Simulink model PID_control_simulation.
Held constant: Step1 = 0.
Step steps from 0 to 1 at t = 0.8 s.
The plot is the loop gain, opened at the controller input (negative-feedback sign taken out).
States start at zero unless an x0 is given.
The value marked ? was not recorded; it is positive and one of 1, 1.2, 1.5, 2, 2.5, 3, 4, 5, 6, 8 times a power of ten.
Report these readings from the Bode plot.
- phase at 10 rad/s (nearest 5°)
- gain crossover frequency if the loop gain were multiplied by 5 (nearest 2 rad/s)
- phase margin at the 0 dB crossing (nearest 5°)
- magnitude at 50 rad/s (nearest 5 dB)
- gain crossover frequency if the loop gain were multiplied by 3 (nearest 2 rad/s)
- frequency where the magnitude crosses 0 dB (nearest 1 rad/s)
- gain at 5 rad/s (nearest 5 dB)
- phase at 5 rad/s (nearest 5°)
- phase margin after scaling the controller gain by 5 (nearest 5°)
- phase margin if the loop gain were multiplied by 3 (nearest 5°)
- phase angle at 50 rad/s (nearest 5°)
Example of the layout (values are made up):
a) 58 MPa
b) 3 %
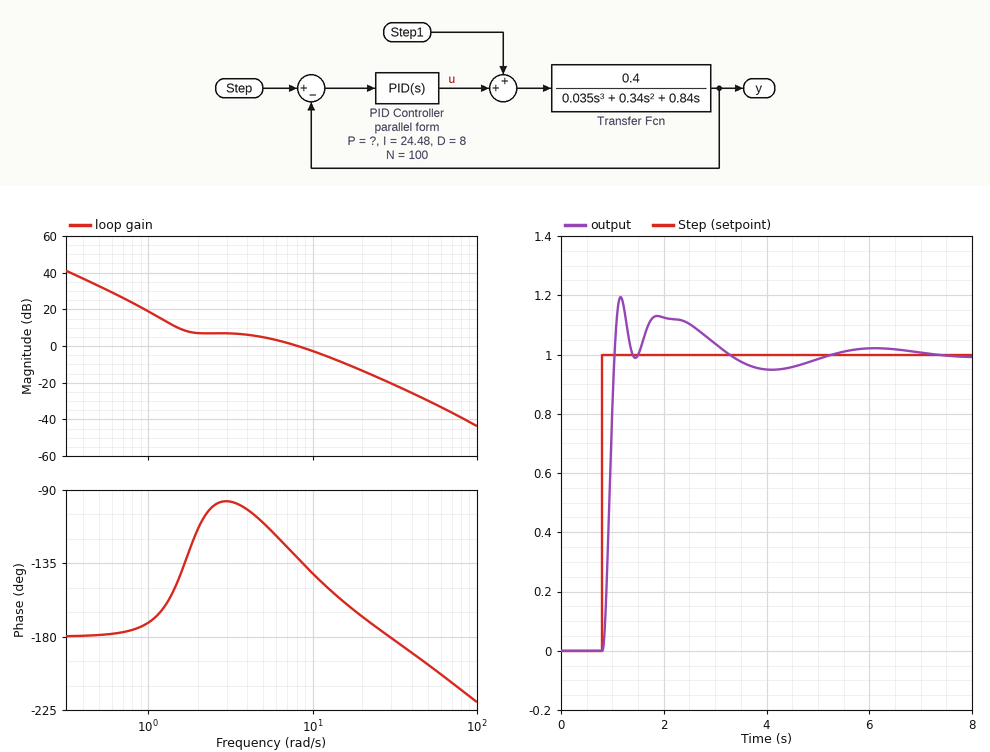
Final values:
a) -140°
b) 20 rad/s
c) 50°
d) -30 dB
e) 16 rad/s
f) 8 rad/s
g) 5 dB
h) -110°
i) 10°
j) 20°
k) -195°
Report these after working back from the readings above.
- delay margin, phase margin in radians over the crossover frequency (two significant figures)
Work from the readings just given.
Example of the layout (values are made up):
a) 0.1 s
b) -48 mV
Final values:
a) 0.11 s
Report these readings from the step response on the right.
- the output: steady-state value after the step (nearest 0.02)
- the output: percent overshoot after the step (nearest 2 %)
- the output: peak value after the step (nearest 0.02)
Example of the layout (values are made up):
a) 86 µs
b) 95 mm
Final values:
a) 1.00
b) 20 %
c) 1.20
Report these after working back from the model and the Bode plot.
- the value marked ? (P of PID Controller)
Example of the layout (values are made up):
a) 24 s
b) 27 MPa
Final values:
a) 10
